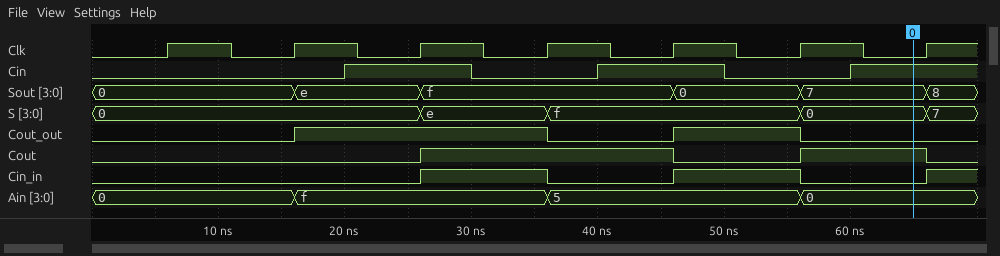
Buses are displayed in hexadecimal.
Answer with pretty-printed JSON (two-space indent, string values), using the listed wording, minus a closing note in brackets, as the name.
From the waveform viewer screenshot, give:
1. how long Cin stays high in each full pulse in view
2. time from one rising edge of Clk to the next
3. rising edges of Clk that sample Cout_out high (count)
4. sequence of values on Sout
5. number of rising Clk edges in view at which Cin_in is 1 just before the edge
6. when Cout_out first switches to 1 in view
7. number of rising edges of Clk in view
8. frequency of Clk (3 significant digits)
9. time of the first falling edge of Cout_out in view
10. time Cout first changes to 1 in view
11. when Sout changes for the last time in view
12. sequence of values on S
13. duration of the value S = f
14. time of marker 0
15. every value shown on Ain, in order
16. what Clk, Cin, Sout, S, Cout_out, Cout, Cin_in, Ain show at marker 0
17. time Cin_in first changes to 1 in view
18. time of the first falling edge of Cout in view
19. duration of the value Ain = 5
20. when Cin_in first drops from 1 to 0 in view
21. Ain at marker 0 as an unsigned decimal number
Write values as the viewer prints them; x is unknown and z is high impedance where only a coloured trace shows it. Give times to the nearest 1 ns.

{
  "how long Cin stays high in each full pulse in view": "10 ns, 10 ns",
  "time from one rising edge of Clk to the next": "10 ns",
  "rising edges of Clk that sample Cout_out high": "3",
  "sequence of values on Sout": "0, e, f, 0, 7, 8",
  "number of rising Clk edges in view at which Cin_in is 1 just before the edge": "2",
  "when Cout_out first switches to 1 in view": "16 ns",
  "number of rising edges of Clk in view": "7",
  "frequency of Clk": "100 MHz",
  "time of the first falling edge of Cout_out in view": "36 ns",
  "time Cout first changes to 1 in view": "26 ns",
  "when Sout changes for the last time in view": "66 ns",
  "sequence of values on S": "0, e, f, 0, 7",
  "duration of the value S = f": "20 ns",
  "time of marker 0": "65 ns",
  "every value shown on Ain, in order": "0, f, 5, 0",
  "what Clk, Cin, Sout, S, Cout_out, Cout, Cin_in, Ain show at marker 0": "Clk=0, Cin=1, Sout=7, S=0, Cout_out=0, Cout=1, Cin_in=0, Ain=0",
  "time Cin_in first changes to 1 in view": "26 ns",
  "time of the first falling edge of Cout in view": "46 ns",
  "duration of the value Ain = 5": "20 ns",
  "when Cin_in first drops from 1 to 0 in view": "36 ns",
  "Ain at marker 0 as an unsigned decimal number": "0"
}
